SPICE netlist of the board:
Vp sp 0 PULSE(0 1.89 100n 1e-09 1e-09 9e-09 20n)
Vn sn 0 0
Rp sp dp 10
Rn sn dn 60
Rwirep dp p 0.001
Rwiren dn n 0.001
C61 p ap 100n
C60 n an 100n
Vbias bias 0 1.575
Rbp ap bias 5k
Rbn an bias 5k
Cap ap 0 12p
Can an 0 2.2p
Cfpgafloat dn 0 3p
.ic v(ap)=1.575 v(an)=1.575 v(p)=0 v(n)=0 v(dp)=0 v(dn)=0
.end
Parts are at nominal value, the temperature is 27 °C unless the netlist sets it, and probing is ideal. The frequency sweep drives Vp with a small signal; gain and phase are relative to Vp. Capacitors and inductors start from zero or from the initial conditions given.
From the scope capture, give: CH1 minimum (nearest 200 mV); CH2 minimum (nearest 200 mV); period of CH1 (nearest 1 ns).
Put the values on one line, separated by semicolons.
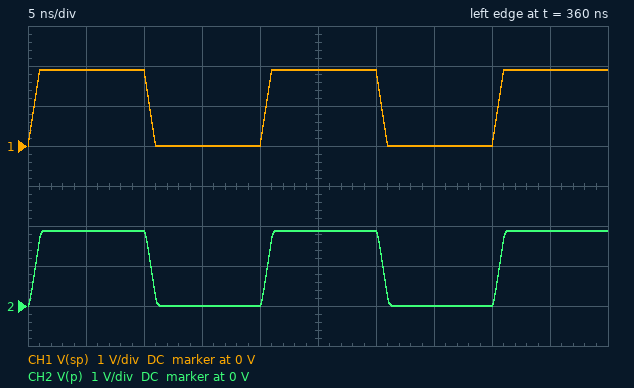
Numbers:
0 V; 0 V; 20 ns
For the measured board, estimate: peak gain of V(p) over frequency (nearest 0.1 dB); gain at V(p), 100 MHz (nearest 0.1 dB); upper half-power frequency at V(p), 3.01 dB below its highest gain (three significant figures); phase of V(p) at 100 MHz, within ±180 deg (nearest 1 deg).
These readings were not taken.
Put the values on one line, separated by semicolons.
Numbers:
0 dB; 0 dB; 1.33 GHz; -4 deg
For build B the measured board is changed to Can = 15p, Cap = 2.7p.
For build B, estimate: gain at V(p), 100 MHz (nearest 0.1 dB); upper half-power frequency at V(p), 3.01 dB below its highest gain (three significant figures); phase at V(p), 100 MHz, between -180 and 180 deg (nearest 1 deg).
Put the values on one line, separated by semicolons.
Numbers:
0 dB; 5.91 GHz; -1 deg
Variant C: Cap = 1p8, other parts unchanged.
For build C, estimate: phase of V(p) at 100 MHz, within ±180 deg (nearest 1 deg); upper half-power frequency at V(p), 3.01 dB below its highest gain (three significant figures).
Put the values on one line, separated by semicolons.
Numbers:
-1 deg; 8.86 GHz
